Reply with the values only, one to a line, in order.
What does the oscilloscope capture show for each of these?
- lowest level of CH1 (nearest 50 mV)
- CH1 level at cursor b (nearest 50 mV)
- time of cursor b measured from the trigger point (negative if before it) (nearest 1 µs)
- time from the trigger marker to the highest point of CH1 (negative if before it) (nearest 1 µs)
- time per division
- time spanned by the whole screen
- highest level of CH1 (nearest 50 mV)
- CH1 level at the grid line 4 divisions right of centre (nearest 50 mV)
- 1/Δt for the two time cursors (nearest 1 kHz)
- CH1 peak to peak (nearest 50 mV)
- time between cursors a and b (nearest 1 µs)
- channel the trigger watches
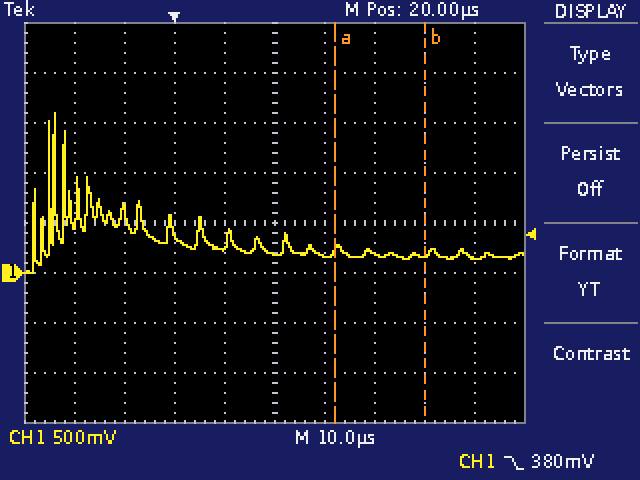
0 mV
200 mV
+50 µs
-24 µs
10 µs
100 µs
1.60 V
150 mV
56 kHz
1.60 V
18 µs
CH1
